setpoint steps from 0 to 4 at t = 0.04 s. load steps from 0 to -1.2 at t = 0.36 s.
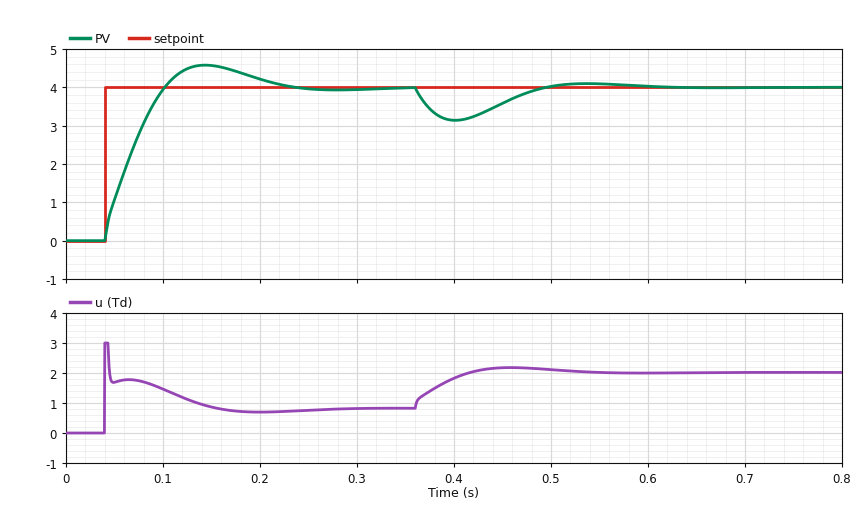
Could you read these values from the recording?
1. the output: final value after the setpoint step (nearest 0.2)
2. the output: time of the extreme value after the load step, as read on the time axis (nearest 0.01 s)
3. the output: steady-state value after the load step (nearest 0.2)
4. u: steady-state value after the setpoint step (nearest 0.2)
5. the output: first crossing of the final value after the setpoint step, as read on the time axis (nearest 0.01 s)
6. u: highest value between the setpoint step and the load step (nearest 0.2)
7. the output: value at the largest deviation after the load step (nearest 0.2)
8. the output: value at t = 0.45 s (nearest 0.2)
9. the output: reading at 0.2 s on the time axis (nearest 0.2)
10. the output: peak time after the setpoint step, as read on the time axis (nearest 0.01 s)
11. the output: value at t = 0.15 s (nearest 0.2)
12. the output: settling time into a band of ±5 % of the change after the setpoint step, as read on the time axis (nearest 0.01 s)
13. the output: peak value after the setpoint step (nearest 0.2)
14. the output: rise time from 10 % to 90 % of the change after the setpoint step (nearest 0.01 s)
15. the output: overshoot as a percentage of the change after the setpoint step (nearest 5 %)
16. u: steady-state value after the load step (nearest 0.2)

4.0
0.40 s
4.0
0.8
0.10 s
3.0
3.2
3.6
4.2
0.14 s
4.6
0.20 s
4.6
0.05 s
15 %
2.0
